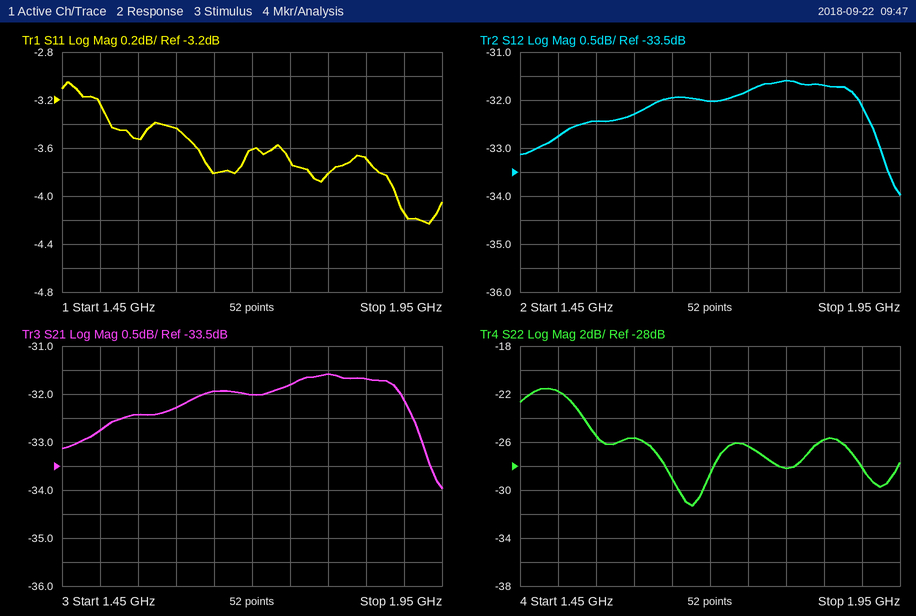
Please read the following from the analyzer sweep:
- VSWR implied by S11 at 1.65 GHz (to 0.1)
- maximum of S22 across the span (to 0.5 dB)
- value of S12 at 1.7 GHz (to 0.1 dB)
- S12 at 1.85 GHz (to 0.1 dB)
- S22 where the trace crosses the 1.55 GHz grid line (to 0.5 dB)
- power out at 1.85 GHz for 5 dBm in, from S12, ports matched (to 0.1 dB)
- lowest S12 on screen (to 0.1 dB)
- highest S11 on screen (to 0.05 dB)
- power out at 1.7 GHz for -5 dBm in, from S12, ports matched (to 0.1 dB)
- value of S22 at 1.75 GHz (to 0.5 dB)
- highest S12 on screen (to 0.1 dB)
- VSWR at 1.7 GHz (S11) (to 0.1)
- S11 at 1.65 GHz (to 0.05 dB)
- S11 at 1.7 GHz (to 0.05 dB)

4.6
-21.5 dB
-32.0 dB
-31.7 dB
-25.5 dB
-26.7 dBm
-34.0 dB
-3.05 dB
-37.0 dBm
-26.5 dB
-31.6 dB
4.9
-3.80 dB
-3.60 dB
